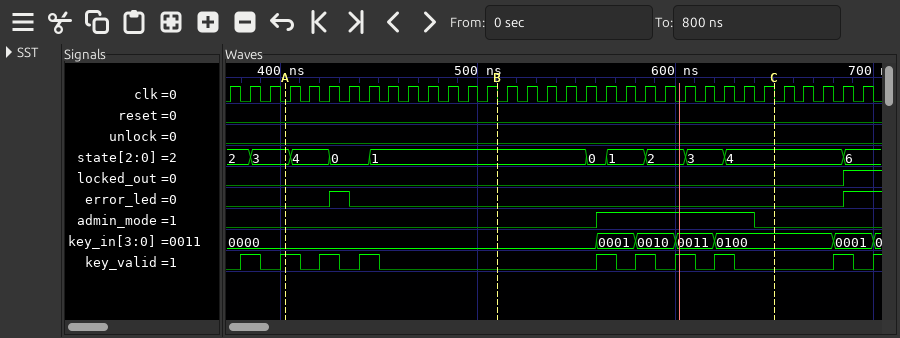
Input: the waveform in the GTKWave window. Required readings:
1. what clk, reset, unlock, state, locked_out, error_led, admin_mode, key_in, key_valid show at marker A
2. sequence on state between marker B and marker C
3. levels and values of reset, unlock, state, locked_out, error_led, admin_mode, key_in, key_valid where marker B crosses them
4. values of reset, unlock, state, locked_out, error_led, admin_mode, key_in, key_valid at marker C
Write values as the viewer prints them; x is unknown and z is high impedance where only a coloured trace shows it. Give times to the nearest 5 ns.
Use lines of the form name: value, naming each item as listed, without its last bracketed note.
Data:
what clk, reset, unlock, state, locked_out, error_led, admin_mode, key_in, key_valid show at marker A: clk=0, reset=0, unlock=0, state=3, locked_out=0, error_led=0, admin_mode=0, key_in=0000, key_valid=1
sequence on state between marker B and marker C: 1, 0, 1, 2, 3, 4
levels and values of reset, unlock, state, locked_out, error_led, admin_mode, key_in, key_valid where marker B crosses them: reset=0, unlock=0, state=1, locked_out=0, error_led=0, admin_mode=0, key_in=0000, key_valid=0
values of reset, unlock, state, locked_out, error_led, admin_mode, key_in, key_valid at marker C: reset=0, unlock=0, state=4, locked_out=0, error_led=0, admin_mode=0, key_in=0100, key_valid=0
